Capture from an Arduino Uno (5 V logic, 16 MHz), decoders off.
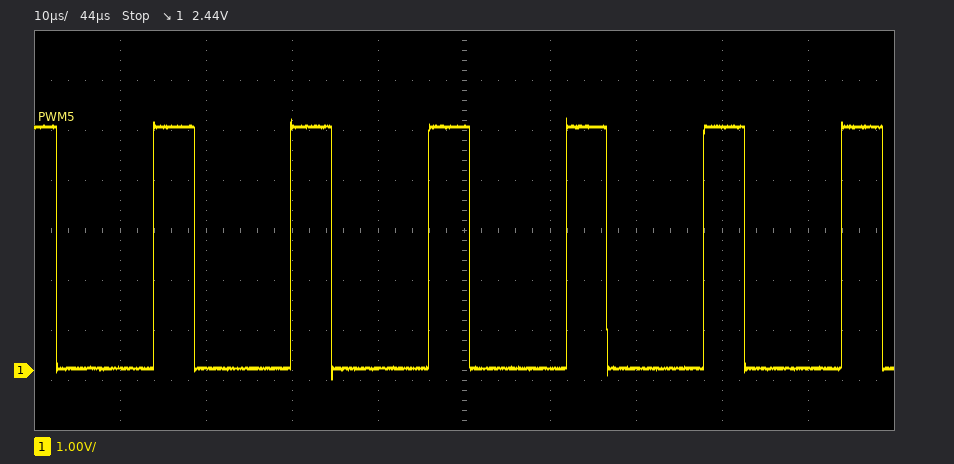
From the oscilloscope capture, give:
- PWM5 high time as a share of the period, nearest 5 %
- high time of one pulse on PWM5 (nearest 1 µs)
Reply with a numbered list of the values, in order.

1. 30 %
2. 5 µs
